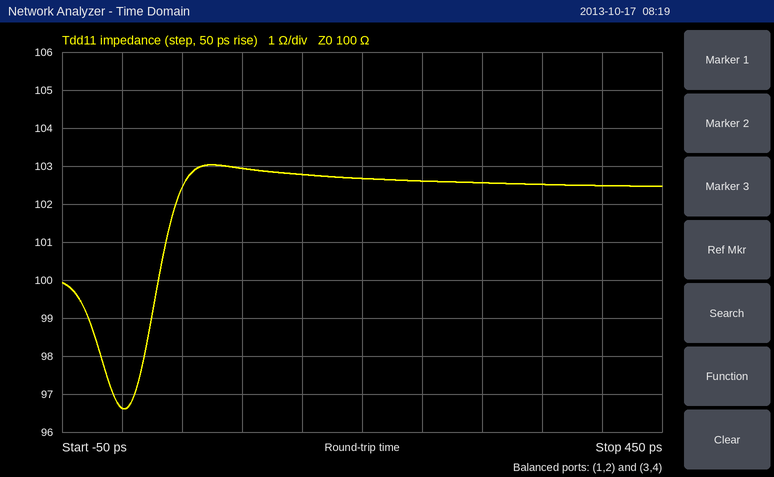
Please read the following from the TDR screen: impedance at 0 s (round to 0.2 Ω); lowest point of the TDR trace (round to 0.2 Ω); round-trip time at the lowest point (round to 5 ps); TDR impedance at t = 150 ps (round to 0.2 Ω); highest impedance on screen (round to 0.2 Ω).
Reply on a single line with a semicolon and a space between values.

96.6 Ω; 96.6 Ω; 0 ps; 102.8 Ω; 103.0 Ω
